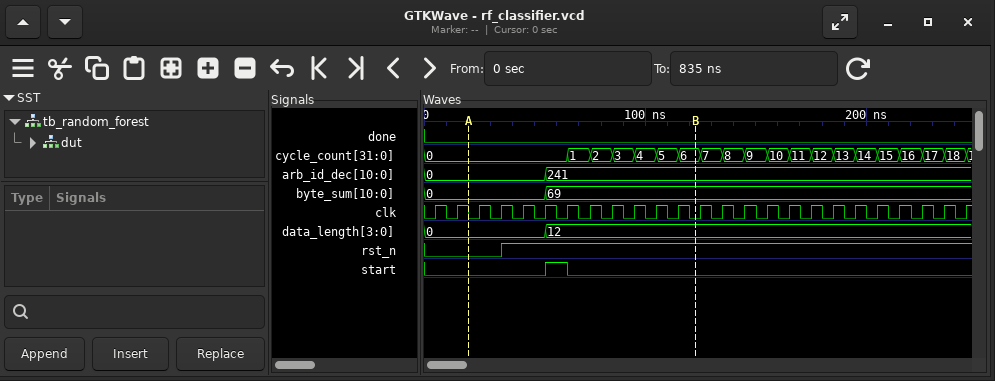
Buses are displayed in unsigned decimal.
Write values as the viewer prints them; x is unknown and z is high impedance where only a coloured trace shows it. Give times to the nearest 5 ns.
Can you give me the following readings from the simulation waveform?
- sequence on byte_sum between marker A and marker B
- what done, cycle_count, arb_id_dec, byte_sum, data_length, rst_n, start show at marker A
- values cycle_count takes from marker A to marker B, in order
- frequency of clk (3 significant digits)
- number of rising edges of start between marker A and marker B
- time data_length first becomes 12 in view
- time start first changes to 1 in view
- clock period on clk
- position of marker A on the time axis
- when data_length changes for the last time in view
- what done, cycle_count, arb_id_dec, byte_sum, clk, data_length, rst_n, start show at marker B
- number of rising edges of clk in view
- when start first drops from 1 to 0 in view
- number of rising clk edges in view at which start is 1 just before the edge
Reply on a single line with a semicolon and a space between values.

0, 69; done=0, cycle_count=0, arb_id_dec=0, byte_sum=0, data_length=0, rst_n=0, start=0; 0, 1, 2, 3, 4, 5, 6; 100 MHz; 1; 55 ns; 55 ns; 10 ns; 20 ns; 55 ns; done=0, cycle_count=6, arb_id_dec=241, byte_sum=69, clk=0, data_length=12, rst_n=1, start=0; 25; 65 ns; 1
